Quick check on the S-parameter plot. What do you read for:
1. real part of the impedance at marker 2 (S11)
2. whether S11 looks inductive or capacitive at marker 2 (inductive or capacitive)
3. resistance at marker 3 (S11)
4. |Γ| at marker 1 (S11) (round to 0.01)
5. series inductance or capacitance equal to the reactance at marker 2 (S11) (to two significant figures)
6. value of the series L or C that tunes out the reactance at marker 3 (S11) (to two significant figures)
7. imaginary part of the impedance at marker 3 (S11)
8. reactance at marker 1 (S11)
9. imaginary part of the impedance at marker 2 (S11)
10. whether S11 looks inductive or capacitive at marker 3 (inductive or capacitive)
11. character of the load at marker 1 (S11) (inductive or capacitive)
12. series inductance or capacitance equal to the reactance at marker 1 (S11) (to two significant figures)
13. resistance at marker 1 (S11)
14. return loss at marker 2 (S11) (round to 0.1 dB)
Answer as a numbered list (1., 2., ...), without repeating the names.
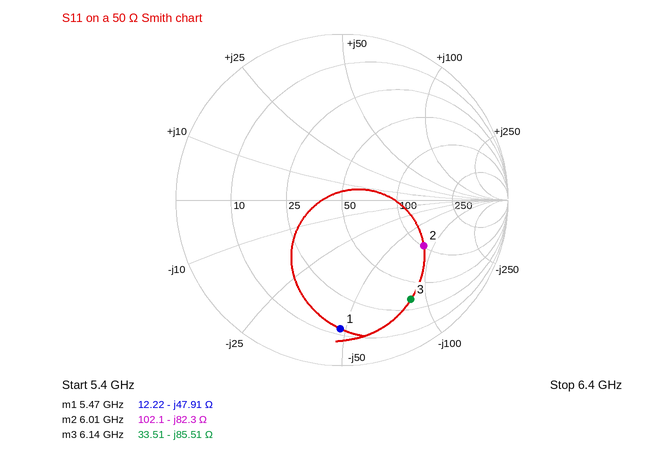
1. 102.1 Ω
2. capacitive
3. 33.51 Ω
4. 0.78
5. 320 fF
6. 2.2 nH
7. -85.51 Ω
8. -47.91 Ω
9. -82.3 Ω
10. capacitive
11. capacitive
12. 610 fF
13. 12.22 Ω
14. 5.0 dB
